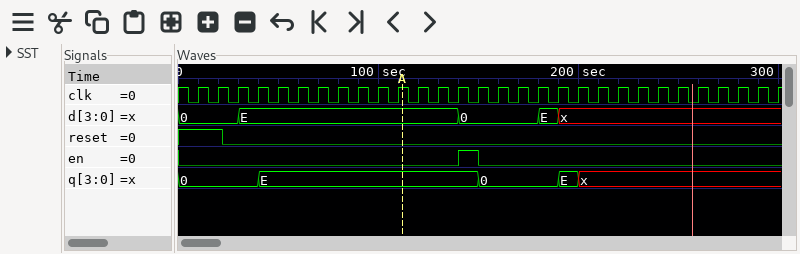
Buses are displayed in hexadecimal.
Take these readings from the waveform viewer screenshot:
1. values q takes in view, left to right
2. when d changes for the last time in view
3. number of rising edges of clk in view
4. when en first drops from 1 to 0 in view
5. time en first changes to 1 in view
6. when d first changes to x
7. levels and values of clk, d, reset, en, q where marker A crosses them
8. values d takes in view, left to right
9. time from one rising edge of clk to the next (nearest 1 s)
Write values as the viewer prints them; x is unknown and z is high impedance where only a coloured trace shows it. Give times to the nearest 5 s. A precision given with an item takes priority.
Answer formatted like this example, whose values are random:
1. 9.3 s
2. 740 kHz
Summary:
1. 0, E, 0, E, x
2. 190 s
3. 30
4. 150 s
5. 140 s
6. 190 s
7. clk=1, d=E, reset=0, en=0, q=E
8. 0, E, 0, E, x
9. 10 s
